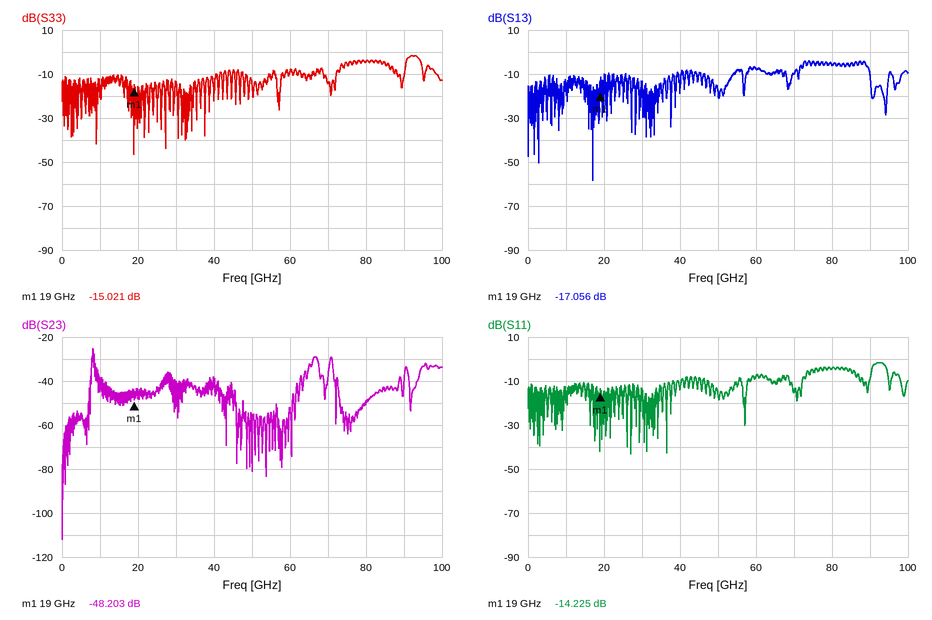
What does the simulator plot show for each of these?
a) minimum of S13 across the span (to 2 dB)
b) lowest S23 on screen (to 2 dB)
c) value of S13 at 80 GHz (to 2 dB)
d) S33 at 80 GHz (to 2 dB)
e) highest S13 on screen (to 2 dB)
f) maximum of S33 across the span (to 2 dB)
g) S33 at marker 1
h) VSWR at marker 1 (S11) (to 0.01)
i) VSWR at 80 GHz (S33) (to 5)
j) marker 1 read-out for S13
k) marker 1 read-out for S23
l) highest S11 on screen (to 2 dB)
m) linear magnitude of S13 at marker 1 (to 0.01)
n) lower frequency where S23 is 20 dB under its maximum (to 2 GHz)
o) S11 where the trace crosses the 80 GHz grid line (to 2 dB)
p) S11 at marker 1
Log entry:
-58 dB
-112 dB
-6 dB
-4 dB
-4 dB
-2 dB
-15.021 dB
1.48
5
-17.056 dB
-48.203 dB
-2 dB
0.14
8 GHz
-4 dB
-14.225 dB
